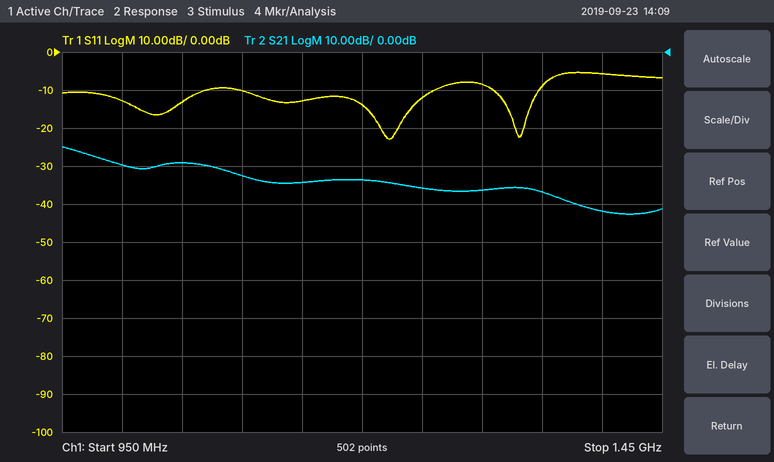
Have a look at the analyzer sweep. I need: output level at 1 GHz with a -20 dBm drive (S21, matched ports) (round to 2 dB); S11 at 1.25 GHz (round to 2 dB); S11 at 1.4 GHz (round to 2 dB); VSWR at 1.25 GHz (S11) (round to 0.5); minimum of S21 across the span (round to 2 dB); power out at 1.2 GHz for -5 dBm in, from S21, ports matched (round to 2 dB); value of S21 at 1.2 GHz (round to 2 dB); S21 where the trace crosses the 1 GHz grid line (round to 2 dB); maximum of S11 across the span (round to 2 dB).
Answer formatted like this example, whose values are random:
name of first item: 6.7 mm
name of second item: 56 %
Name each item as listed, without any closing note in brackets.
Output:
output level at 1 GHz with a -20 dBm drive (S21, matched ports): -50 dBm
S11 at 1.25 GHz: -12 dB
S11 at 1.4 GHz: -6 dB
VSWR at 1.25 GHz (S11): 1.5
minimum of S21 across the span: -42 dB
power out at 1.2 GHz for -5 dBm in, from S21, ports matched: -38 dBm
value of S21 at 1.2 GHz: -34 dB
S21 where the trace crosses the 1 GHz grid line: -30 dB
maximum of S11 across the span: -6 dB
